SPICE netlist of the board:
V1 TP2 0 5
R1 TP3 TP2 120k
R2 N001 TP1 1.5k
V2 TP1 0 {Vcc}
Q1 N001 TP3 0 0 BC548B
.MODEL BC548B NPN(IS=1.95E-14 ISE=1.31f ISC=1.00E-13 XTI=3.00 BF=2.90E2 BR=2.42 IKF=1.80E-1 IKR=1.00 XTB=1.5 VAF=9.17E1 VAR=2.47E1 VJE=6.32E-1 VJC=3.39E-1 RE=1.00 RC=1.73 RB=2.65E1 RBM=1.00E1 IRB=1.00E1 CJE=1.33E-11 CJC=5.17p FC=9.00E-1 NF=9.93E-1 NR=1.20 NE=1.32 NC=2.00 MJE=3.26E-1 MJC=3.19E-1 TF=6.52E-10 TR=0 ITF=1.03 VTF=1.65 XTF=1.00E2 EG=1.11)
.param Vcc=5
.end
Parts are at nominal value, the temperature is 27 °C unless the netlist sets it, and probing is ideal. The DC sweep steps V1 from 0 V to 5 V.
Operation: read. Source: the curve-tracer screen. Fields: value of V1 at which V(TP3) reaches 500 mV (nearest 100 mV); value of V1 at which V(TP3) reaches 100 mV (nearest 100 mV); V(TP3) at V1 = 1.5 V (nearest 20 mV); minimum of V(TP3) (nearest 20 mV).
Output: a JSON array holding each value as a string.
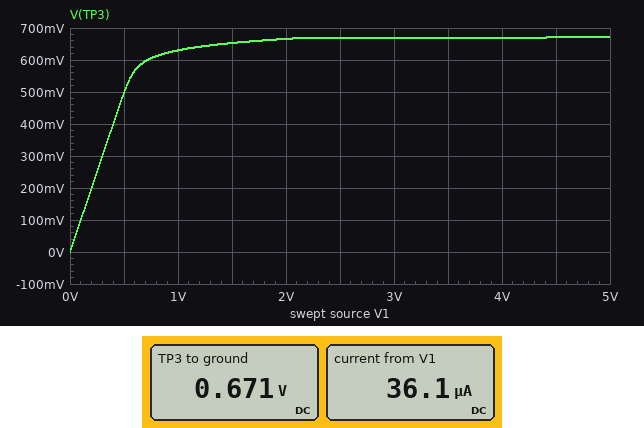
["500 mV", "100 mV", "660 mV", "0 V"]
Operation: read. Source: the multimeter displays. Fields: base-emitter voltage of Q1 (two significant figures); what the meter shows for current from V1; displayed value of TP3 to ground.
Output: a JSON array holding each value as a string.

["670 mV", "36.1 µA", "0.671 V"]
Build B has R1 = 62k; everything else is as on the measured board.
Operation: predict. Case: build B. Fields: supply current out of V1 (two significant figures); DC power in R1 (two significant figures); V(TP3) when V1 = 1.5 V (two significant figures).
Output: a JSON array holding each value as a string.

["70 µA", "300 µW", "670 mV"]
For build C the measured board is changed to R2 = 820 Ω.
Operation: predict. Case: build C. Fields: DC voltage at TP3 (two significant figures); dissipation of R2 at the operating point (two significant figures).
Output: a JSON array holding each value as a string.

["690 mV", "30 mW"]
